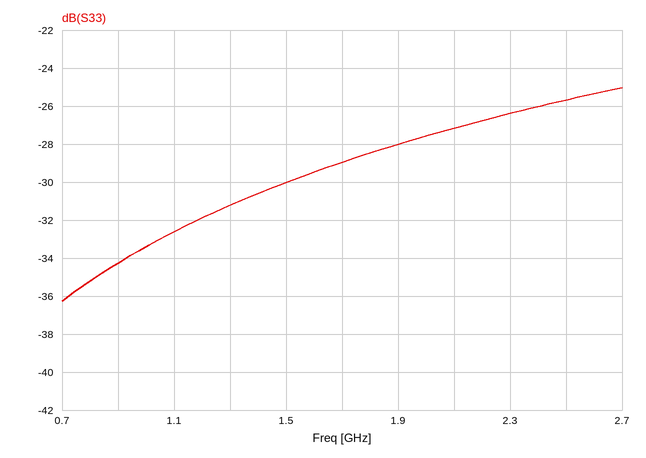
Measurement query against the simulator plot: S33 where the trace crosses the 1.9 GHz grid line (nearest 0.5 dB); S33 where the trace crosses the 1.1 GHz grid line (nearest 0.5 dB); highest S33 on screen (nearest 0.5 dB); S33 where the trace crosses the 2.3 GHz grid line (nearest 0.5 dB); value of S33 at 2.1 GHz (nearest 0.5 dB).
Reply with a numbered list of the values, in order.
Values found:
1. -28.0 dB
2. -32.5 dB
3. -25.0 dB
4. -26.5 dB
5. -27.0 dB
